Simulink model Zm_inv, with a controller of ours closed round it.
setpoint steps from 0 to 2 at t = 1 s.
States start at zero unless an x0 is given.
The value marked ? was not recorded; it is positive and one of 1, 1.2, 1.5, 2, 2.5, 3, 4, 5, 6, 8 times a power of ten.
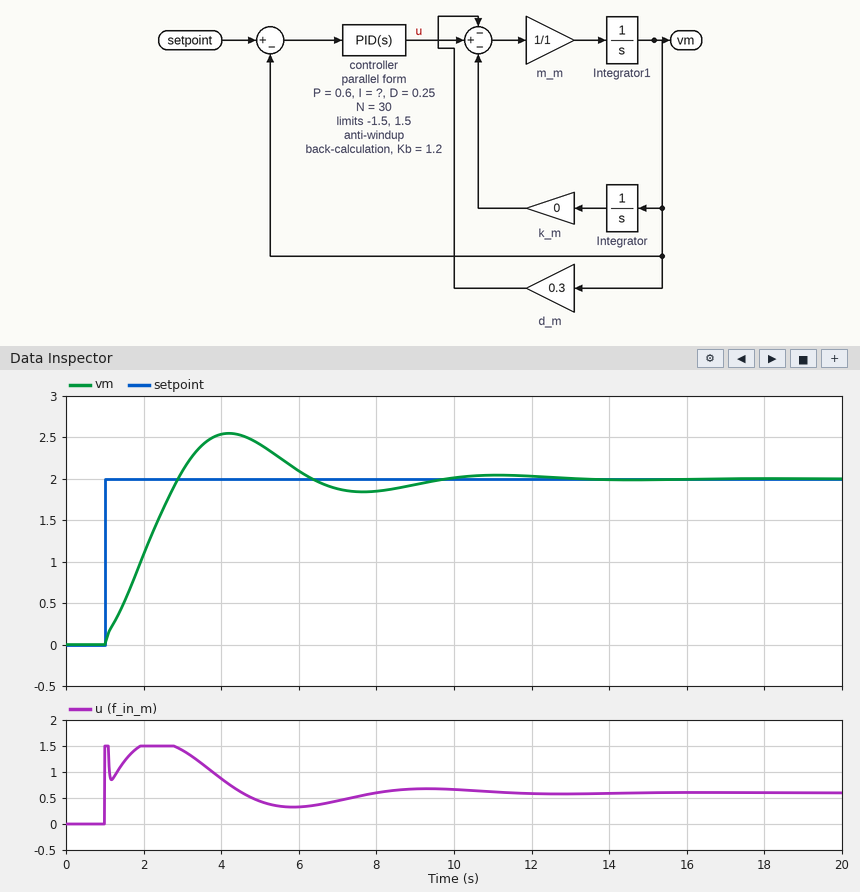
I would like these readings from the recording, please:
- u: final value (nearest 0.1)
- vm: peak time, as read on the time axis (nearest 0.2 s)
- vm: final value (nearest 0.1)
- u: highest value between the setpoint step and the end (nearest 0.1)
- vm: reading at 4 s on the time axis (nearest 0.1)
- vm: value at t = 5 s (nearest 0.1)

0.6
4.2 s
2.0
1.5
2.5
2.4
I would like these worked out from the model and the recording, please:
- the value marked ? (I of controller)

1.2
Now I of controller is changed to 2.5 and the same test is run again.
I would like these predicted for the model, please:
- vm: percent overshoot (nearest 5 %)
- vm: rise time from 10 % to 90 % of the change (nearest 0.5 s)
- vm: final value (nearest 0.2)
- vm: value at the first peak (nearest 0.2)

30 %
1.5 s
2.0
2.6
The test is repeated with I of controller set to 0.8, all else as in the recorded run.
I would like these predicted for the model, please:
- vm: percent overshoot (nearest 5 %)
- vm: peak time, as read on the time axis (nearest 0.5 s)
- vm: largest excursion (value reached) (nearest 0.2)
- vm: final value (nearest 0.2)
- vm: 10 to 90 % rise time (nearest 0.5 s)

20 %
5.0 s
2.4
2.0
2.0 s
